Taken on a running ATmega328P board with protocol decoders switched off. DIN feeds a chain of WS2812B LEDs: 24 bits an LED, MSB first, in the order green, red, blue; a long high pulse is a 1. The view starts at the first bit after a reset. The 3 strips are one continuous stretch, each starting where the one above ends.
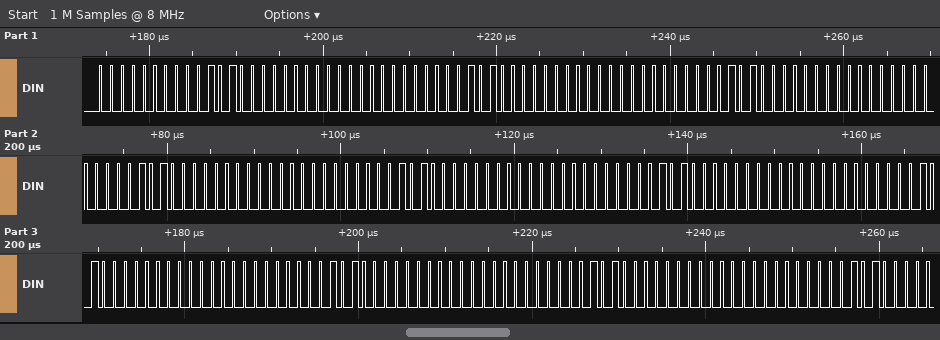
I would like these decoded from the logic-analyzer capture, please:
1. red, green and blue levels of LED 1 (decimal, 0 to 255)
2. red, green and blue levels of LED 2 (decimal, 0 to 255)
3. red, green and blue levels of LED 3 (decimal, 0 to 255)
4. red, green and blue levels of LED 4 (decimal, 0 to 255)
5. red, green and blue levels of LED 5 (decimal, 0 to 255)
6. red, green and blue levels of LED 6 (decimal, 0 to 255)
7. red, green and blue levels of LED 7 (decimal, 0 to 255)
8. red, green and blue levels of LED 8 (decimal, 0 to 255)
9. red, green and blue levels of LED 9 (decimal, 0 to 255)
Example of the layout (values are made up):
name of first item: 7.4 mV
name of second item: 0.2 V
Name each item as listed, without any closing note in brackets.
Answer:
red, green and blue levels of LED 1: 40, 0, 0
red, green and blue levels of LED 2: 40, 0, 0
red, green and blue levels of LED 3: 40, 0, 0
red, green and blue levels of LED 4: 40, 0, 0
red, green and blue levels of LED 5: 40, 0, 0
red, green and blue levels of LED 6: 40, 0, 0
red, green and blue levels of LED 7: 40, 0, 0
red, green and blue levels of LED 8: 40, 0, 0
red, green and blue levels of LED 9: 40, 0, 0
